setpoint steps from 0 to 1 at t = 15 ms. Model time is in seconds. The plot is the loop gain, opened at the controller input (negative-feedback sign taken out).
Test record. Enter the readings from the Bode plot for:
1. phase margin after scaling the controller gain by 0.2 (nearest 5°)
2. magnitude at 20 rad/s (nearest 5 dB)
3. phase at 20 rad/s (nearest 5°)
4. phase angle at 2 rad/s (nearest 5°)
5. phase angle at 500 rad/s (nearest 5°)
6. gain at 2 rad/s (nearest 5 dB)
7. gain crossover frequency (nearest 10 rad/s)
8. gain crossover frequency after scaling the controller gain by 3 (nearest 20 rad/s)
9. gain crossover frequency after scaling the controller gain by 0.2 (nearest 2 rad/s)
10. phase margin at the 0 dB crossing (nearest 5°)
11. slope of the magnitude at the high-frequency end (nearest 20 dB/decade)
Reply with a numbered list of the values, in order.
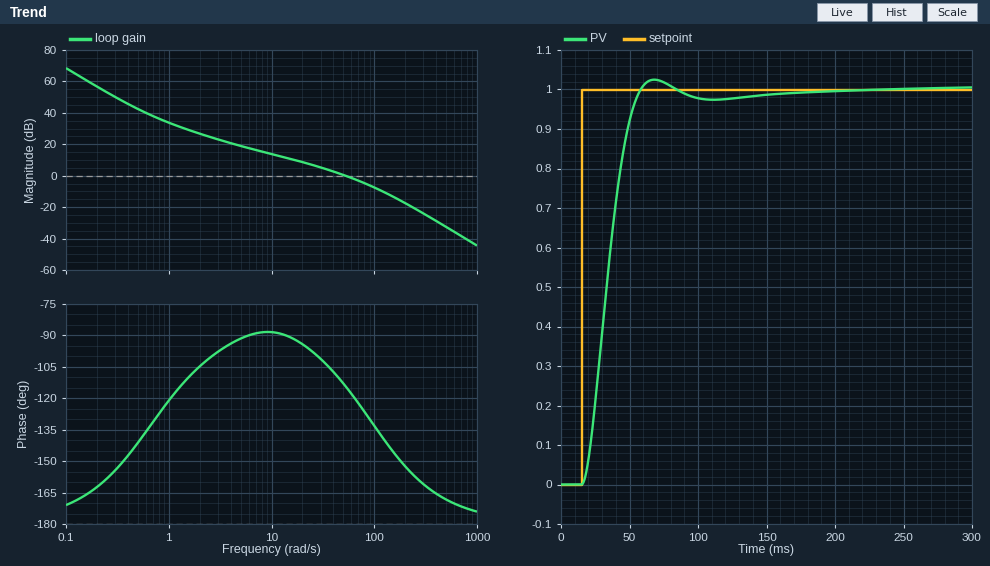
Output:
1. 90°
2. 10 dB
3. -95°
4. -105°
5. -170°
6. 25 dB
7. 50 rad/s
8. 120 rad/s
9. 10 rad/s
10. 65°
11. -40 dB/decade
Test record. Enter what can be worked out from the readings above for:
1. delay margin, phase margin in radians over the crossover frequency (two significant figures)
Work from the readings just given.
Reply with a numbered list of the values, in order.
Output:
1. 0.023 s
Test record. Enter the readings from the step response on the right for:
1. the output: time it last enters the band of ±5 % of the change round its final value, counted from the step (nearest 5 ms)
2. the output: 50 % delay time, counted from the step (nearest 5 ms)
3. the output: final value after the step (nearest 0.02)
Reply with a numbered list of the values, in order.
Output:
1. 40 ms
2. 20 ms
3. 1.00
